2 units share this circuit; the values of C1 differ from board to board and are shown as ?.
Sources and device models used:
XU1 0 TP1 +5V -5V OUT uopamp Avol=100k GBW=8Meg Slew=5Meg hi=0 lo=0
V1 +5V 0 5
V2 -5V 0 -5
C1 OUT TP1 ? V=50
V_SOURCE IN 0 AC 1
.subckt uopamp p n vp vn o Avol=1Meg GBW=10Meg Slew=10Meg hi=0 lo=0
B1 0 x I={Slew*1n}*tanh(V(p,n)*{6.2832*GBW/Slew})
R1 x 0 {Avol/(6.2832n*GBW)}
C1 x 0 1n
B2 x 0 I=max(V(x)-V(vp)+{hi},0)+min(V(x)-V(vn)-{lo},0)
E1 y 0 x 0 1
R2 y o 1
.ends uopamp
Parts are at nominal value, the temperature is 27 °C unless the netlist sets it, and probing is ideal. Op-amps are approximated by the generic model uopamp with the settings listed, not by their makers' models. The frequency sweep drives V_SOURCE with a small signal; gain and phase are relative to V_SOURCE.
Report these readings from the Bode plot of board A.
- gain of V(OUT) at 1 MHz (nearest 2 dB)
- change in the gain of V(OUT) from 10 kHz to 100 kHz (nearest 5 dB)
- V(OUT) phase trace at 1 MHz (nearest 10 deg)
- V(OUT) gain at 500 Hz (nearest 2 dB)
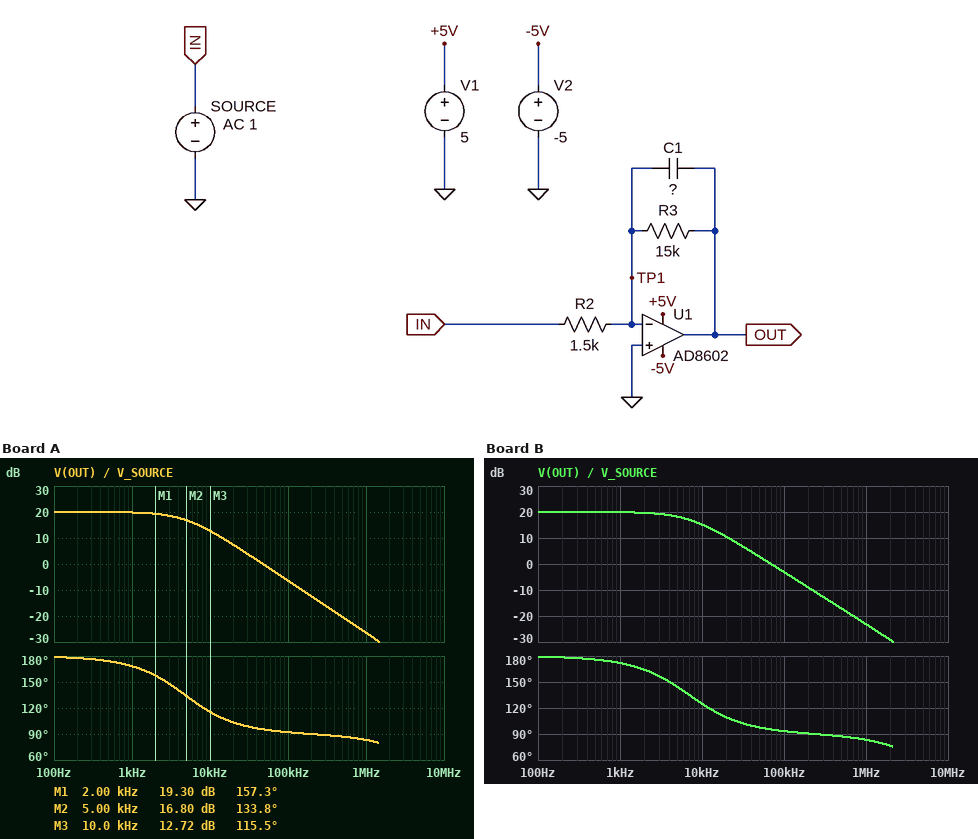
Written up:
-26 dB
-20 dB
80 deg
20 dB
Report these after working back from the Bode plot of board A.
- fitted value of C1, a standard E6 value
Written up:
2.2 nF
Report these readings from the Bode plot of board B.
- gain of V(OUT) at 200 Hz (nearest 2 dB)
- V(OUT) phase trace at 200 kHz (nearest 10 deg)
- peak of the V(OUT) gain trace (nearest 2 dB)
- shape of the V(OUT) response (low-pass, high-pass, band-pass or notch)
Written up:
20 dB
90 deg
20 dB
low-pass
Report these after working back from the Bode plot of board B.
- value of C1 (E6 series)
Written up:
1.5 nF
